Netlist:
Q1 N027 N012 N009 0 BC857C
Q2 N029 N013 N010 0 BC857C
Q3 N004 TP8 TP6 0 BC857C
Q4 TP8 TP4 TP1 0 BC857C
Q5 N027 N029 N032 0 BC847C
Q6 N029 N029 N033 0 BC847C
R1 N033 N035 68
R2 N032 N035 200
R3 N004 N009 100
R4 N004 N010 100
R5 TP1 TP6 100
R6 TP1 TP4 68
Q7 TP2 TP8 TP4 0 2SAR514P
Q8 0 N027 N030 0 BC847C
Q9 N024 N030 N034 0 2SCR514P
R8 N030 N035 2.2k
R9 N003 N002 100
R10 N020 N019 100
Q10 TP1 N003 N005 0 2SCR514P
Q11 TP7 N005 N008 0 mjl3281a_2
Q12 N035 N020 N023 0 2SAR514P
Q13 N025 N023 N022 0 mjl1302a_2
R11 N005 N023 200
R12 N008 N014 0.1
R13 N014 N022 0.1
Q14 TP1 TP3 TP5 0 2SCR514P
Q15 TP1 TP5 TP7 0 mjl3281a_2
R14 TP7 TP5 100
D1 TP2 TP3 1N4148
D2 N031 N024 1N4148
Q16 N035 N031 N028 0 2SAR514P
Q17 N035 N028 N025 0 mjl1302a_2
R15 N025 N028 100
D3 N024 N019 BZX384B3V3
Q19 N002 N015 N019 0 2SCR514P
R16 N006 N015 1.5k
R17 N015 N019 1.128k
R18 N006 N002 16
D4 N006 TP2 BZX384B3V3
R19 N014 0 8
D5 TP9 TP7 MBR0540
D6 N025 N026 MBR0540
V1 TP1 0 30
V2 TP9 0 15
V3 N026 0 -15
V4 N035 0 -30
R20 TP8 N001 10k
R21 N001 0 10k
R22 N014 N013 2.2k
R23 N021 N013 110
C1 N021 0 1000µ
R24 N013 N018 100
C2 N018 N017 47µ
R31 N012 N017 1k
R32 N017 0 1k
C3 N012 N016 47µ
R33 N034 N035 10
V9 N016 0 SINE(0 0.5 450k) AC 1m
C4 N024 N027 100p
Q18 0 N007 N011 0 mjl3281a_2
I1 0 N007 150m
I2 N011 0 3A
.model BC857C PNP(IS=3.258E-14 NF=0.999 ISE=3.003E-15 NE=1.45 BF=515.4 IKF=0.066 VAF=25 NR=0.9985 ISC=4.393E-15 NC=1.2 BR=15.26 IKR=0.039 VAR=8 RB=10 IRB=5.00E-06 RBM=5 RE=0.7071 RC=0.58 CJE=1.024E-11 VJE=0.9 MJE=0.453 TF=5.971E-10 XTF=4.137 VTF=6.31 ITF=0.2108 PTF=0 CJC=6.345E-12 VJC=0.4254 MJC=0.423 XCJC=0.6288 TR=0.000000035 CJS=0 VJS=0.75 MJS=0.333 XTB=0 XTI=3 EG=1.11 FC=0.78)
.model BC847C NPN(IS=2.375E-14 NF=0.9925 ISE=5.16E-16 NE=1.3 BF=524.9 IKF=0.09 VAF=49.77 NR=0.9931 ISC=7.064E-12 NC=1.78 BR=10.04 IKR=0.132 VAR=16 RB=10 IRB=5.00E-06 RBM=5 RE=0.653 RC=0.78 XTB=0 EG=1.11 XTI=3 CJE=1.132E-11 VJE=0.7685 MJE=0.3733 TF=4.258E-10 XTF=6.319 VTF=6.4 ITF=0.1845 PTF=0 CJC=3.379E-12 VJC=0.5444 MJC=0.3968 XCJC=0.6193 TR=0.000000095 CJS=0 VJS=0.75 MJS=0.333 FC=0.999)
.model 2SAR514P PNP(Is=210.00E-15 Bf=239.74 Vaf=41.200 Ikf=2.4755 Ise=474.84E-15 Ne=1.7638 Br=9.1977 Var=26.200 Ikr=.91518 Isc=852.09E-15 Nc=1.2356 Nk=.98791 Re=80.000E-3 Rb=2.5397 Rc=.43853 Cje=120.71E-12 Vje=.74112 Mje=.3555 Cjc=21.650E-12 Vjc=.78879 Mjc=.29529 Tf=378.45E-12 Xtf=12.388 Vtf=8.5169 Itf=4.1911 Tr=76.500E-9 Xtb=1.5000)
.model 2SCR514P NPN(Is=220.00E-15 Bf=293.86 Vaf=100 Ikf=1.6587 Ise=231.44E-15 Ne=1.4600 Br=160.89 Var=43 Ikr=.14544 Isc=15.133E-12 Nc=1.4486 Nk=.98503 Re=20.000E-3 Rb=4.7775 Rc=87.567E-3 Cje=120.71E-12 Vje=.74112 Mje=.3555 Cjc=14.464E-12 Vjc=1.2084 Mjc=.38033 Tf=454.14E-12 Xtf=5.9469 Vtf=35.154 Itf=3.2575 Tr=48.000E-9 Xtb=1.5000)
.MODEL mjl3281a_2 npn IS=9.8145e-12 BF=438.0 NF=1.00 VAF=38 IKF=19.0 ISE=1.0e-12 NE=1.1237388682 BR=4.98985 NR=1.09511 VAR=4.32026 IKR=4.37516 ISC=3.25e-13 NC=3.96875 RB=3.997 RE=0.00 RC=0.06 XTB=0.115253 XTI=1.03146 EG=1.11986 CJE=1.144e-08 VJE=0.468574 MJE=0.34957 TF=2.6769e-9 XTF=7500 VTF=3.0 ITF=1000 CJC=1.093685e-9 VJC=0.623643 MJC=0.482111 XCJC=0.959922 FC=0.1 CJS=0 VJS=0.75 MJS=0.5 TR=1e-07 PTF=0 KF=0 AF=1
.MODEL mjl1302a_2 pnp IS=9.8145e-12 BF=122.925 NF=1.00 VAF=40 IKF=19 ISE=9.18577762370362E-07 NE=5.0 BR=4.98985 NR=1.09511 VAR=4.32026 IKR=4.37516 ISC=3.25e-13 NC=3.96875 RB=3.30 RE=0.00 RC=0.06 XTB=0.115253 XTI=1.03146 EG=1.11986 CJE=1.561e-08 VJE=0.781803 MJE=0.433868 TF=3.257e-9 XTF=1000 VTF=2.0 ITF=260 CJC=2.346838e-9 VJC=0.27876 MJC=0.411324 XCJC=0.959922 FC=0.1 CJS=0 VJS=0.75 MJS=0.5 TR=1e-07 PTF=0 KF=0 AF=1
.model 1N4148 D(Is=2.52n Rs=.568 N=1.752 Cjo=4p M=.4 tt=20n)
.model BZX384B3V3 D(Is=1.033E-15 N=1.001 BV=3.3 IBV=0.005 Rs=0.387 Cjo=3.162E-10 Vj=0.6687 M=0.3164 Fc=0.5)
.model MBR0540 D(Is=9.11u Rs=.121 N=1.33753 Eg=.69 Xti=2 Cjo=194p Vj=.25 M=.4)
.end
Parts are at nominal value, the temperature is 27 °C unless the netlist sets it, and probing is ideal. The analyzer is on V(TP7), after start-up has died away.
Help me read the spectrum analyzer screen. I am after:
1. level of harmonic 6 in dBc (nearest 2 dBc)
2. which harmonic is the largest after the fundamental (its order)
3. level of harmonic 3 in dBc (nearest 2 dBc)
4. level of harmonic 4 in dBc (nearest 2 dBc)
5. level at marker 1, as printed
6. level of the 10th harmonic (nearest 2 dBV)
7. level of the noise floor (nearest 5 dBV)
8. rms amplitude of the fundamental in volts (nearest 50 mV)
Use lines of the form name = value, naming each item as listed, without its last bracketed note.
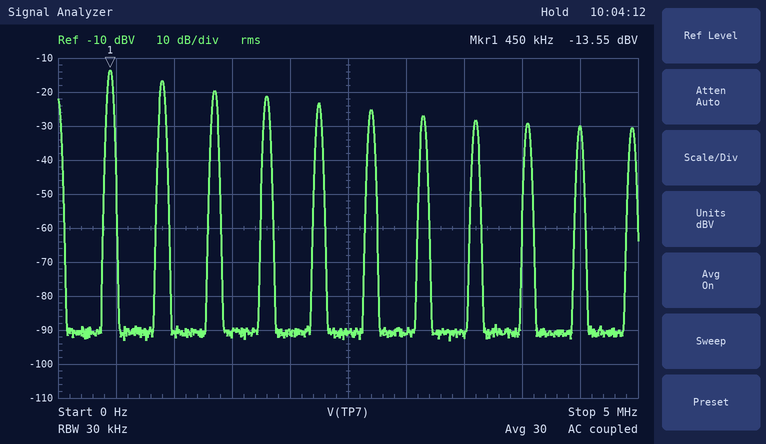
level of harmonic 6 in dBc = -12 dBc
which harmonic is the largest after the fundamental = 2
level of harmonic 3 in dBc = -6 dBc
level of harmonic 4 in dBc = -8 dBc
level at marker 1, as printed = -13.55 dBV
level of the 10th harmonic = -30 dBV
level of the noise floor = -90 dBV
rms amplitude of the fundamental in volts = 200 mV
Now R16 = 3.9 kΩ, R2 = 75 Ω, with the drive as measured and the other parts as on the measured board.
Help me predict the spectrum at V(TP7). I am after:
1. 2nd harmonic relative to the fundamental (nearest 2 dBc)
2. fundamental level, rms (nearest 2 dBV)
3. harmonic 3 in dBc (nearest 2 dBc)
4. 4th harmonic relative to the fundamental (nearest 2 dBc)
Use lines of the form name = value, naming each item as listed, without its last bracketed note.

2nd harmonic relative to the fundamental = -18 dBc
fundamental level, rms = -22 dBV
harmonic 3 in dBc = -36 dBc
4th harmonic relative to the fundamental = -34 dBc
